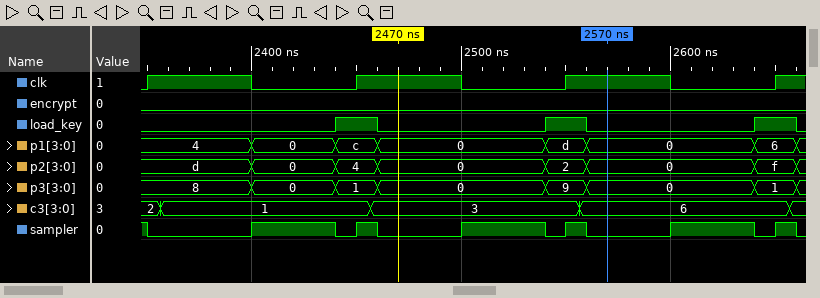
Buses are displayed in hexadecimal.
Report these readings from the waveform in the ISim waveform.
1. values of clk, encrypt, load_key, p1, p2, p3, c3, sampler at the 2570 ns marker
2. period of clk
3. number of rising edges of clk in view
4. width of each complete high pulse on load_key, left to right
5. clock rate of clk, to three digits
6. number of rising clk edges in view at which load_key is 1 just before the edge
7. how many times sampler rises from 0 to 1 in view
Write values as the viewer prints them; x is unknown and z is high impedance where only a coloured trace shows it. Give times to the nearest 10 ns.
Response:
clk=1, encrypt=0, load_key=0, p1=0, p2=0, p3=0, c3=6, sampler=0
100 ns
4
20 ns, 20 ns, 20 ns
10.0 MHz
3
6
